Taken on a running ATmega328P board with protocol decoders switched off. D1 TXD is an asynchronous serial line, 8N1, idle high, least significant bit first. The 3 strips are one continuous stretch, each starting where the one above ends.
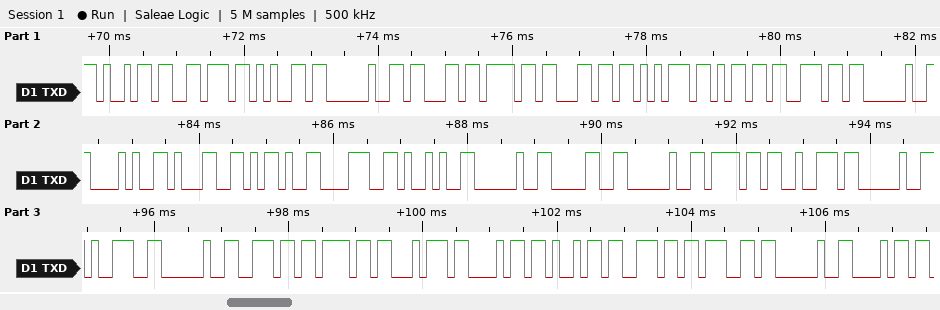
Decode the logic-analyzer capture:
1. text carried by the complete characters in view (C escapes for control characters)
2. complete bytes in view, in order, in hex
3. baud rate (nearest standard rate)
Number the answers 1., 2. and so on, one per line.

1. "ive column (1-8) 0 or 9 nothing h"
2. 69 76 65 20 63 6F 6C 75 6D 6E 20 28 31 2D 38 29 20 30 20 6F 72 20 39 20 6E 6F 74 68 69 6E 67 20 68
3. 9600 baud
